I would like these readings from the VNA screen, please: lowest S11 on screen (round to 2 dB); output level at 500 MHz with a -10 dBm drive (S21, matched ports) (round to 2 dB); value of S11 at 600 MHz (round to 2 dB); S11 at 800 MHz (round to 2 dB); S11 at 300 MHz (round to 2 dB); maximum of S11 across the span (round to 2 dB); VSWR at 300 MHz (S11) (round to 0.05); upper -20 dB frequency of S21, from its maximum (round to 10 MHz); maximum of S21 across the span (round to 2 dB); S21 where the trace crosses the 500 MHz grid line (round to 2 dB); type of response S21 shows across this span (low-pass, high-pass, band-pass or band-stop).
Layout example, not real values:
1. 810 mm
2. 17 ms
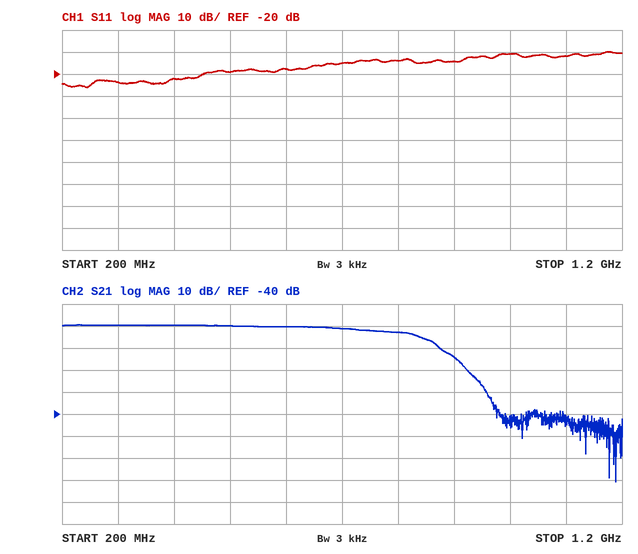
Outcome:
1. -26 dB
2. -10 dBm
3. -18 dB
4. -14 dB
5. -24 dB
6. -10 dB
7. 1.15
8. 920 MHz
9. 0 dB
10. 0 dB
11. low-pass
